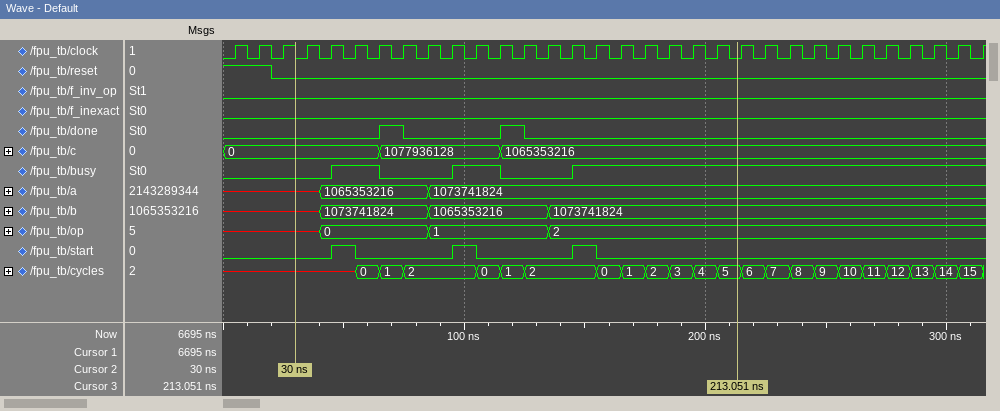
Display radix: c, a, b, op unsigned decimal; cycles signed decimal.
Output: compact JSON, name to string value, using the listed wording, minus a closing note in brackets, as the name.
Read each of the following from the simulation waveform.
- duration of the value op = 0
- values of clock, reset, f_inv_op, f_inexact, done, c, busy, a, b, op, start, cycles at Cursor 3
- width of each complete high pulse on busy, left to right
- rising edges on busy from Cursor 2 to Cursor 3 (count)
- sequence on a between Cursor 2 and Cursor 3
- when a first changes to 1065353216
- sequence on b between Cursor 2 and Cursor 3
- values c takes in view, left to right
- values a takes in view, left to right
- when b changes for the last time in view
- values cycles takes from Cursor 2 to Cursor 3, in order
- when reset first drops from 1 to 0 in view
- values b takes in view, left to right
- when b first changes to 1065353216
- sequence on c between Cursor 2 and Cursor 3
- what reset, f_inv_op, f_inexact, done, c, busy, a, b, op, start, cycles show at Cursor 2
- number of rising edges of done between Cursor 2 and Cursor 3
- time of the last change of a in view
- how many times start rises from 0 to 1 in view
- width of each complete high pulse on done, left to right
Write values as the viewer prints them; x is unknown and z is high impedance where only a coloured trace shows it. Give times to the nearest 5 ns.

{"duration of the value op = 0": "45 ns", "values of clock, reset, f_inv_op, f_inexact, done, c, busy, a, b, op, start, cycles at Cursor 3": "clock=0, reset=0, f_inv_op=0, f_inexact=0, done=0, c=1065353216, busy=1, a=1073741824, b=1073741824, op=2, start=0, cycles=5", "width of each complete high pulse on busy, left to right": "20 ns, 20 ns", "rising edges on busy from Cursor 2 to Cursor 3": "3", "sequence on a between Cursor 2 and Cursor 3": "x, 1065353216, 1073741824", "when a first changes to 1065353216": "40 ns", "sequence on b between Cursor 2 and Cursor 3": "x, 1073741824, 1065353216, 1073741824", "values c takes in view, left to right": "0, 1077936128, 1065353216", "values a takes in view, left to right": "x, 1065353216, 1073741824", "when b changes for the last time in view": "135 ns", "values cycles takes from Cursor 2 to Cursor 3, in order": "x, 0, 1, 2, 0, 1, 2, 0, 1, 2, 3, 4, 5", "when reset first drops from 1 to 0 in view": "20 ns", "values b takes in view, left to right": "x, 1073741824, 1065353216, 1073741824", "when b first changes to 1065353216": "85 ns", "sequence on c between Cursor 2 and Cursor 3": "0, 1077936128, 1065353216", "what reset, f_inv_op, f_inexact, done, c, busy, a, b, op, start, cycles show at Cursor 2": "reset=0, f_inv_op=0, f_inexact=0, done=0, c=0, busy=0, a=x, b=x, op=x, start=0, cycles=x", "number of rising edges of done between Cursor 2 and Cursor 3": "2", "time of the last change of a in view": "85 ns", "how many times start rises from 0 to 1 in view": "3", "width of each complete high pulse on done, left to right": "10 ns, 10 ns"}
